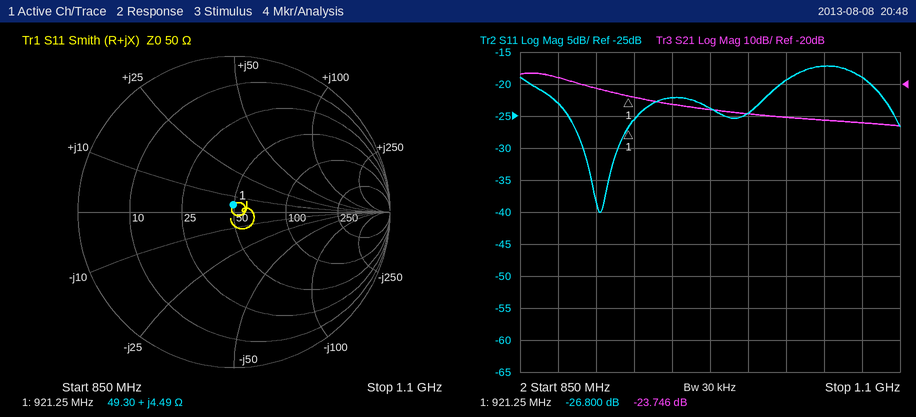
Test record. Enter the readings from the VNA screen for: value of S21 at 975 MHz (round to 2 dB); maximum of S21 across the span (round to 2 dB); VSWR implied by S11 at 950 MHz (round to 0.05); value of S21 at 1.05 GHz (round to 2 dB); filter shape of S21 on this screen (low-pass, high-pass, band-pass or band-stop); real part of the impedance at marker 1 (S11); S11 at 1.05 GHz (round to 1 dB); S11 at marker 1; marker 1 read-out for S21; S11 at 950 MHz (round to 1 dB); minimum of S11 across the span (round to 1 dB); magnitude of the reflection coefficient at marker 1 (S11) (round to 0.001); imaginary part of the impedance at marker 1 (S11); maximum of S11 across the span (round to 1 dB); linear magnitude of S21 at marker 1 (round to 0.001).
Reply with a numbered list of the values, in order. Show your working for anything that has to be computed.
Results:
1. -28 dB
2. -16 dB
3. |Γ| = 10^(-22/20) = 0.0794; VSWR = (1 + 0.0794)/(1 − 0.0794) ≈ 1.17, so 1.15 to the nearest 0.05
4. -32 dB
5. low-pass
6. 49.30 Ω
7. -17 dB
8. -26.800 dB
9. -23.746 dB
10. -22 dB
11. -40 dB
12. 10^(-26.8/20) ≈ 0.046
13. +4.49 Ω
14. -17 dB
15. 10^(-23.746/20) ≈ 0.065
